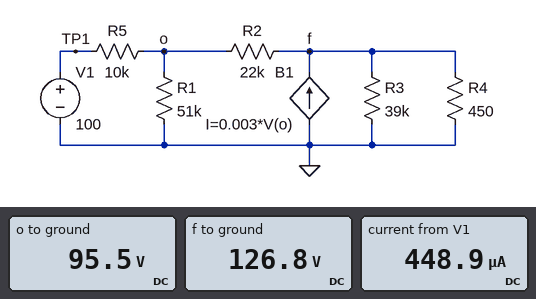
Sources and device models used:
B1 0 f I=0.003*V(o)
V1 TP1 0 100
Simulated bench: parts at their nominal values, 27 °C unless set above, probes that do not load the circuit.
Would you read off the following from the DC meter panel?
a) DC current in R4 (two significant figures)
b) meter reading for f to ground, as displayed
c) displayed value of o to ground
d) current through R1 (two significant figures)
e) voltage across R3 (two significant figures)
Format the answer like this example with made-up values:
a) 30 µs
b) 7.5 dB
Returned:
a) 280 mA
b) 126.8 V
c) 95.5 V
d) 1.9 mA
e) 130 V
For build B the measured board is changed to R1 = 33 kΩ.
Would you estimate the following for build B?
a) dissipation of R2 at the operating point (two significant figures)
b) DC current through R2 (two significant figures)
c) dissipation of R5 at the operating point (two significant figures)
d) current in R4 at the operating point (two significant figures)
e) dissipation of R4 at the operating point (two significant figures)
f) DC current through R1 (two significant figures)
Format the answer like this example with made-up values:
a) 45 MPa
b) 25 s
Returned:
a) 37 mW
b) 1.3 mA
c) 18 mW
d) 260 mA
e) 29 W
f) 2.6 mA
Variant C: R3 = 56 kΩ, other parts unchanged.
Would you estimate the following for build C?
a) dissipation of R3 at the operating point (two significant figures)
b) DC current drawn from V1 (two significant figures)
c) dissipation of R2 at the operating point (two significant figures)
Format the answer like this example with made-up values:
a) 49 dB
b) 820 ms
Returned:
a) 290 mW
b) 430 µA
c) 46 mW
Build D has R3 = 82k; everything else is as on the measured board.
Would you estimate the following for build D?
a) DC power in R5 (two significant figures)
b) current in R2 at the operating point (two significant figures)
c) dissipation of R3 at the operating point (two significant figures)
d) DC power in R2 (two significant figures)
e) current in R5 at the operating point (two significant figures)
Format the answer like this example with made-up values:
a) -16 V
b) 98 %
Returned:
a) 1.7 mW
b) 1.5 mA
c) 200 mW
d) 47 mW
e) 420 µA
